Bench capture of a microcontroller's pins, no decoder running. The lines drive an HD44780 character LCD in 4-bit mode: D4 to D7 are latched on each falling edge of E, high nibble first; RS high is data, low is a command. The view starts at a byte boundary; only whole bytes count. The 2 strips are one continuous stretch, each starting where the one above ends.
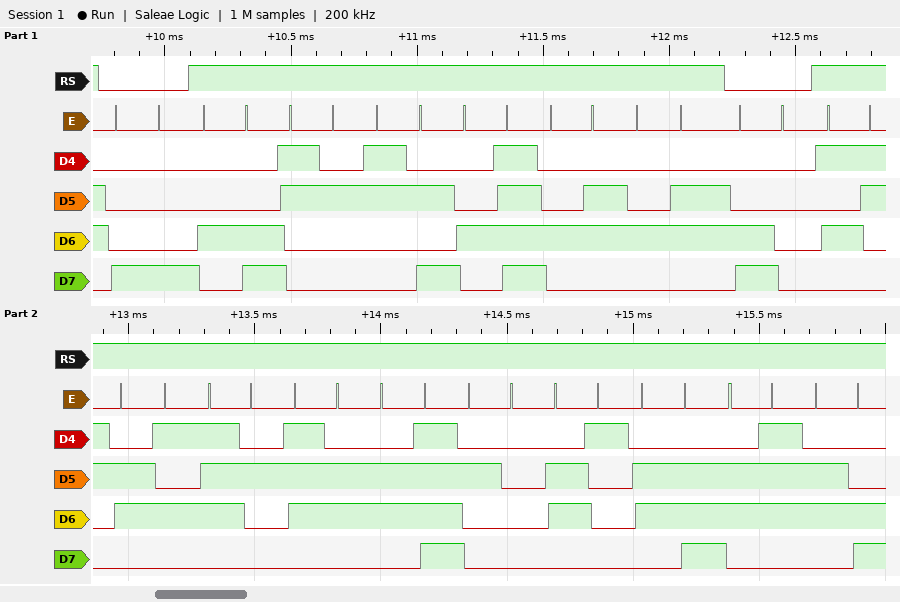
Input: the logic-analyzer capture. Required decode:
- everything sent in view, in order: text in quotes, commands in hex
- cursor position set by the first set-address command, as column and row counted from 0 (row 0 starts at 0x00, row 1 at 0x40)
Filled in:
0x88 "L2:OFF" 0xC0 "Servo angl"
column 8, row 0
